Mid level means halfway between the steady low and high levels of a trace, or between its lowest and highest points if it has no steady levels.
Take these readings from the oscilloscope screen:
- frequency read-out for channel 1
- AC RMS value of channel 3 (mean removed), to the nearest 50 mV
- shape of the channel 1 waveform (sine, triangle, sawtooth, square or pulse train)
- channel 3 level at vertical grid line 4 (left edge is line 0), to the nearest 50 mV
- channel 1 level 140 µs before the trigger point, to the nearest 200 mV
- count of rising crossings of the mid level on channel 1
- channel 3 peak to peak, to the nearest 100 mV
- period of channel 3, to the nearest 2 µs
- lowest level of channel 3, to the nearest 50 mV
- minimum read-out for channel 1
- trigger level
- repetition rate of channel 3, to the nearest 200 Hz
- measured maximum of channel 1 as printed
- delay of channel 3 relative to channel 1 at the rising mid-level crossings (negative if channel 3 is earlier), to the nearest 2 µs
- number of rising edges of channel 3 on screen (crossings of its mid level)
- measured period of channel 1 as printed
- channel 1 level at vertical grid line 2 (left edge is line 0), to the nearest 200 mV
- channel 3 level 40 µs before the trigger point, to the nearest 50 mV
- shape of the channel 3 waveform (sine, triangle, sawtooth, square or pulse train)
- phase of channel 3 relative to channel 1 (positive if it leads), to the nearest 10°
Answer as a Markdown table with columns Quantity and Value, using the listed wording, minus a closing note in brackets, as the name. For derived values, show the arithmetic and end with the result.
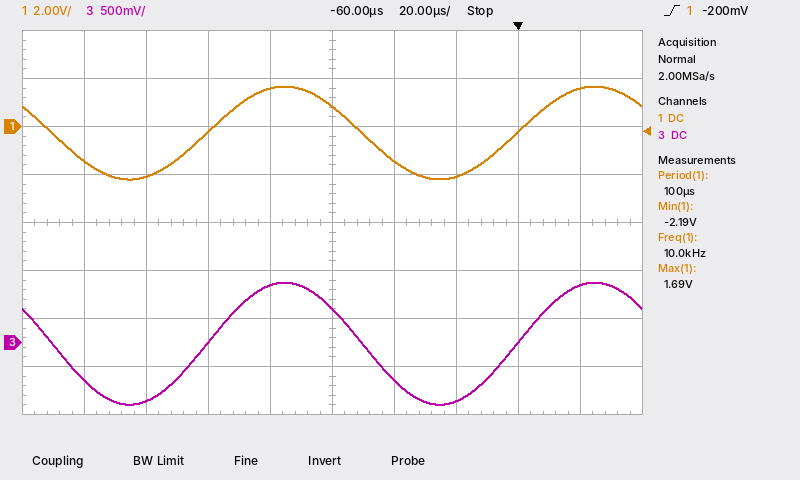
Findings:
| Quantity | Value |
|---|---|
| frequency read-out for channel 1 | 10.0 kHz |
| AC RMS value of channel 3 (mean removed), to the nearest 50 mV | 1.30 V / (2√2) ≈ 460 mV, so 450 mV to the nearest 50 mV |
| shape of the channel 1 waveform | sine |
| channel 3 level at vertical grid line 4 (left edge is line 0), to the nearest 50 mV | 600 mV |
| channel 1 level 140 µs before the trigger point, to the nearest 200 mV | -1.4 V |
| count of rising crossings of the mid level on channel 1 | 2 |
| channel 3 peak to peak, to the nearest 100 mV | 1.30 V |
| period of channel 3, to the nearest 2 µs | 100 µs |
| lowest level of channel 3, to the nearest 50 mV | -650 mV |
| minimum read-out for channel 1 | -2.19 V |
| trigger level | -200 mV |
| repetition rate of channel 3, to the nearest 200 Hz | 1 / 100 µs ≈ 10.0 kHz |
| measured maximum of channel 1 as printed | 1.69 V |
| delay of channel 3 relative to channel 1 at the rising mid-level crossings (negative if channel 3 is earlier), to the nearest 2 µs | 0 µs |
| number of rising edges of channel 3 on screen | 2 |
| measured period of channel 1 as printed | 100 µs |
| channel 1 level at vertical grid line 2 (left edge is line 0), to the nearest 200 mV | -2.0 V |
| channel 3 level 40 µs before the trigger point, to the nearest 50 mV | -400 mV |
| shape of the channel 3 waveform | sine |
| phase of channel 3 relative to channel 1 (positive if it leads), to the nearest 10° | −360° × (0 µs) / 100 µs ≈ 0° |
